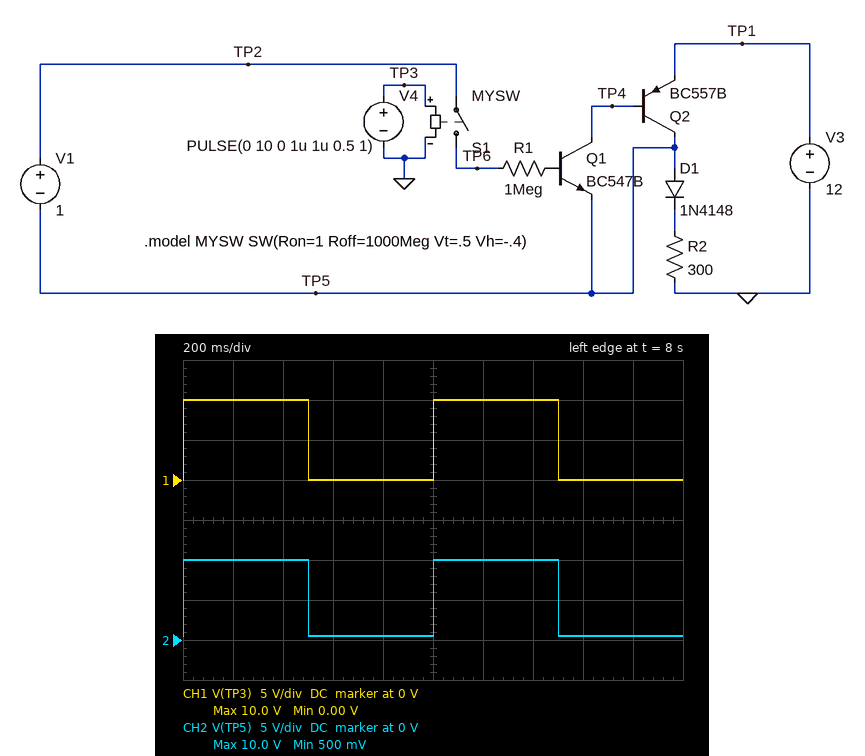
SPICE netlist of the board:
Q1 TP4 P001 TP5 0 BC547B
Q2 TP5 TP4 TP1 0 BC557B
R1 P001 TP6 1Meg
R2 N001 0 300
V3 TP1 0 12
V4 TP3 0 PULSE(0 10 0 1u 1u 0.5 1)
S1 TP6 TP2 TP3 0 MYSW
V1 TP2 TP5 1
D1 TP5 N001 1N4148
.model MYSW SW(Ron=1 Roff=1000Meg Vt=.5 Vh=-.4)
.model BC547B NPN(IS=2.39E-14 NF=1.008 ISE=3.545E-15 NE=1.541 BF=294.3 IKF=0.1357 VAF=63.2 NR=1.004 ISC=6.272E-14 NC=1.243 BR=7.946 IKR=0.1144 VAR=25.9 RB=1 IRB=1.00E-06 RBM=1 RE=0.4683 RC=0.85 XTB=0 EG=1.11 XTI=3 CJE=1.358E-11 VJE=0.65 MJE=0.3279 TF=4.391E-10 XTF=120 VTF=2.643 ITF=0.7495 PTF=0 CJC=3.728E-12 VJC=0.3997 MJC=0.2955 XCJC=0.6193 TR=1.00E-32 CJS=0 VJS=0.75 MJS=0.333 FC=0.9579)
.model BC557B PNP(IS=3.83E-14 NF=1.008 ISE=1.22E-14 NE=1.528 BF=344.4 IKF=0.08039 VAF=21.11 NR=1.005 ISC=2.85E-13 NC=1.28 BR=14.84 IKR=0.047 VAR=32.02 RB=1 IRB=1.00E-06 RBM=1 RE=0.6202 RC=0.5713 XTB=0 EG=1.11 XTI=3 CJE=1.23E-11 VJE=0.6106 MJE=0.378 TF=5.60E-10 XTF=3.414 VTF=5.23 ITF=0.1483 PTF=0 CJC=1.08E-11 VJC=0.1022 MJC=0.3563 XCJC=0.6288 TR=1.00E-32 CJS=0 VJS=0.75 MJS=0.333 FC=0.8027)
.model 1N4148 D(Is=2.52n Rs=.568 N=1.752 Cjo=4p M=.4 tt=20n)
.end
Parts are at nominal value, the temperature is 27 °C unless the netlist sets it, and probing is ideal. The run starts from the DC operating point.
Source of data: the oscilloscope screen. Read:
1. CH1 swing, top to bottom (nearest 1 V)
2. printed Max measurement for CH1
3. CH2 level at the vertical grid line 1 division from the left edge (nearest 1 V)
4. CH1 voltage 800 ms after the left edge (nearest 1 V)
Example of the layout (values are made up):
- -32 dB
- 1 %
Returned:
- 10 V
- 10.0 V
- 10 V
- 0 V
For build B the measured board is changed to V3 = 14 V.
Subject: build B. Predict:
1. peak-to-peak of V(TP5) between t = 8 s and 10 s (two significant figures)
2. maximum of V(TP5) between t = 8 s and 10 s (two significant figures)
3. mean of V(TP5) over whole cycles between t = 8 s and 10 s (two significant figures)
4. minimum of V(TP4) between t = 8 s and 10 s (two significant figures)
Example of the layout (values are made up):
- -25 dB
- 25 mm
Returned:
- 10 V
- 11 V
- 5.6 V
- 13 V
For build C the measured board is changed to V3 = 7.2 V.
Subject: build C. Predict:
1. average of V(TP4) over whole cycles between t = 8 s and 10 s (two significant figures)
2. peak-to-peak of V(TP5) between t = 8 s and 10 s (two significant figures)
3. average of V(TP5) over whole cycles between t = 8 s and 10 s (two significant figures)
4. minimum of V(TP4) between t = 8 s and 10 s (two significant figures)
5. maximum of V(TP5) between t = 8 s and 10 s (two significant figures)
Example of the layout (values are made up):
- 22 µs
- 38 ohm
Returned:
- 6.6 V
- 5.9 V
- 3.4 V
- 6.5 V
- 6.4 V
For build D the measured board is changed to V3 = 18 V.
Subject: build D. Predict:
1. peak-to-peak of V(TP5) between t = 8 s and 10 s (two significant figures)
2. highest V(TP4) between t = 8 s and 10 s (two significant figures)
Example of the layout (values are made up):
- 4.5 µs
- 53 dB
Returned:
- 12 V
- 17 V
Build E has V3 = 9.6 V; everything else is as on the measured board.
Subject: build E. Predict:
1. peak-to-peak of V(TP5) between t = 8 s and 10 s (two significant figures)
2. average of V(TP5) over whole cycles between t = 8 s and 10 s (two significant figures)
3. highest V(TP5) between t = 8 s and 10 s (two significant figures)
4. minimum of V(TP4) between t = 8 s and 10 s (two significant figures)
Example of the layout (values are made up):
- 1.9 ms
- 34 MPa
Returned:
- 8.2 V
- 4.6 V
- 8.7 V
- 8.9 V
